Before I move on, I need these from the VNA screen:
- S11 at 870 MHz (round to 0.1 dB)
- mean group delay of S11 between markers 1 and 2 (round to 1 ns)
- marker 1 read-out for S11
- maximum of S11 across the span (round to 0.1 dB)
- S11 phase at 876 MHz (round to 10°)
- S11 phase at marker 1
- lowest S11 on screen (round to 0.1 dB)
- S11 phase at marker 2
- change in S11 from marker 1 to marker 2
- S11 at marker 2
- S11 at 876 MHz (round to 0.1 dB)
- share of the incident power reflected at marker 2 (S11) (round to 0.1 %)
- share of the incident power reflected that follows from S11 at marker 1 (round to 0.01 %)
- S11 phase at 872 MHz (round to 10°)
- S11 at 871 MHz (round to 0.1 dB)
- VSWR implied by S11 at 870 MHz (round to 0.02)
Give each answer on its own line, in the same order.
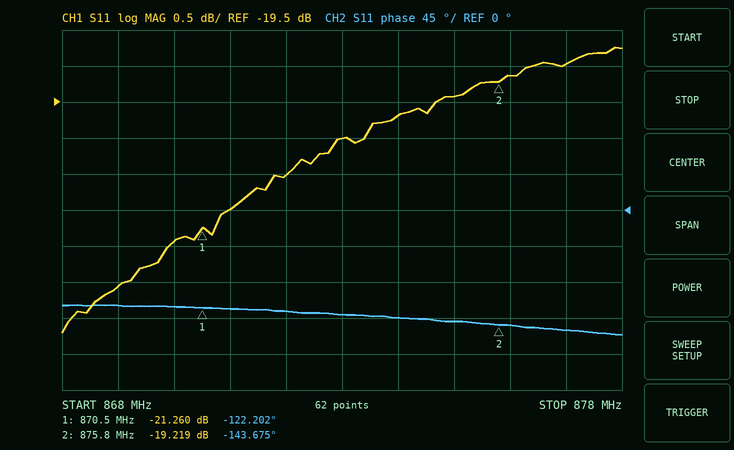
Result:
-21.4 dB
11 ns
-21.260 dB
-18.7 dB
-140°
-122.202°
-22.7 dB
-143.675°
2.041 dB
-19.219 dB
-19.1 dB
1.2 %
0.75 %
-130°
-21.0 dB
1.18
